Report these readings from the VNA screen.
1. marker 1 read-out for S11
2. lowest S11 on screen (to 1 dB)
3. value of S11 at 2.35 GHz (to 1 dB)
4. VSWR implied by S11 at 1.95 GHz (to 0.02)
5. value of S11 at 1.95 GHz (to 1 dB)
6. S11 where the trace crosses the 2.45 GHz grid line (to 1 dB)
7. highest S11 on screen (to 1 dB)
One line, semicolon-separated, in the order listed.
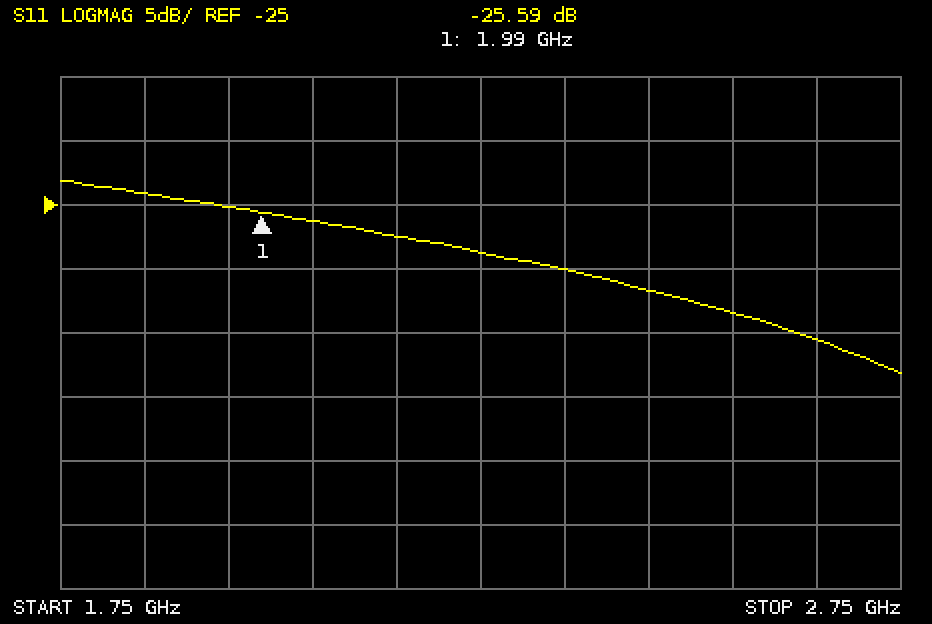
-25.59 dB; -38 dB; -30 dB; 1.12; -25 dB; -32 dB; -23 dB
